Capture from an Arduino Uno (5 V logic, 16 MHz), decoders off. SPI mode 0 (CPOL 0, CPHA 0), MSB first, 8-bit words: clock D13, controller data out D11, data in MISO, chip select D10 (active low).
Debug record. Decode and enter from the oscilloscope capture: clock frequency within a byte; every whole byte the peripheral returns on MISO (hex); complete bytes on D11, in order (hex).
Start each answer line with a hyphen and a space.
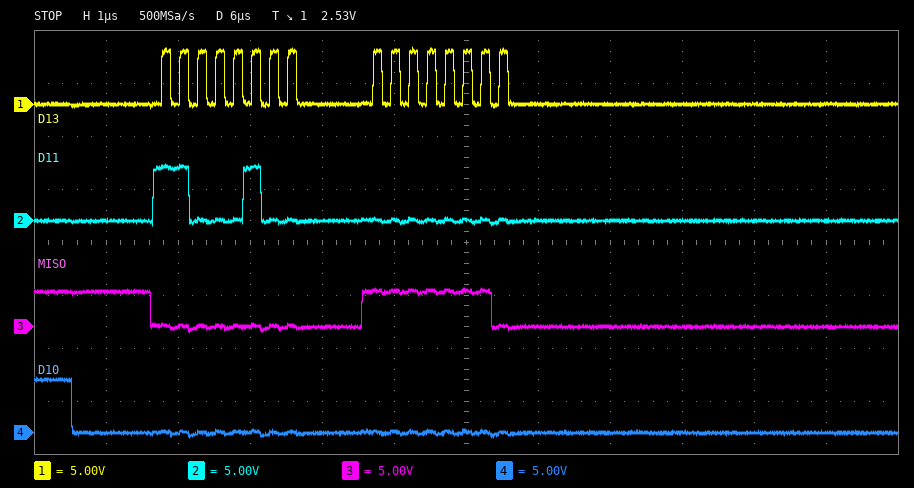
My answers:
- 4 MHz
- 00 FE
- C4 00
